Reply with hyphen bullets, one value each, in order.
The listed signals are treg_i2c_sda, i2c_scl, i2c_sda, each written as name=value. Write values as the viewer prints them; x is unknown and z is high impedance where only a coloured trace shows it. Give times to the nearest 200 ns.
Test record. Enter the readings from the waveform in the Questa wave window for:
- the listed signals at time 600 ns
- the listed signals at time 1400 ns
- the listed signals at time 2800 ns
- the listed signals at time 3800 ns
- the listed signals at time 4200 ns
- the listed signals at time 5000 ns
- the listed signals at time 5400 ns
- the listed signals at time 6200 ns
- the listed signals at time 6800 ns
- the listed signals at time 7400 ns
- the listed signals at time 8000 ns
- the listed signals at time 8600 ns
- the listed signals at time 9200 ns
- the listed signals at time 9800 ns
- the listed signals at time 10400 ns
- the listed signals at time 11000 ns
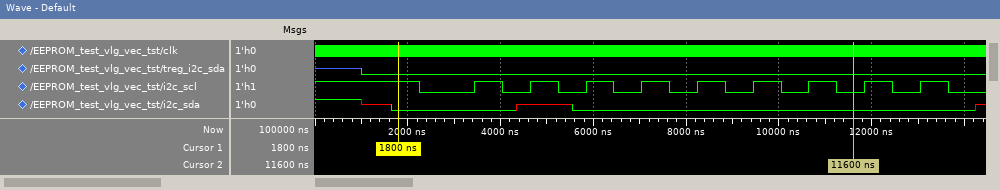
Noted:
- treg_i2c_sda=z, i2c_scl=1, i2c_sda=1
- treg_i2c_sda=0, i2c_scl=1, i2c_sda=x
- treg_i2c_sda=0, i2c_scl=0, i2c_sda=0
- treg_i2c_sda=0, i2c_scl=1, i2c_sda=0
- treg_i2c_sda=0, i2c_scl=0, i2c_sda=0
- treg_i2c_sda=0, i2c_scl=1, i2c_sda=x
- treg_i2c_sda=0, i2c_scl=0, i2c_sda=x
- treg_i2c_sda=0, i2c_scl=1, i2c_sda=0
- treg_i2c_sda=0, i2c_scl=0, i2c_sda=0
- treg_i2c_sda=0, i2c_scl=1, i2c_sda=0
- treg_i2c_sda=0, i2c_scl=0, i2c_sda=0
- treg_i2c_sda=0, i2c_scl=1, i2c_sda=0
- treg_i2c_sda=0, i2c_scl=0, i2c_sda=0
- treg_i2c_sda=0, i2c_scl=1, i2c_sda=0
- treg_i2c_sda=0, i2c_scl=0, i2c_sda=0
- treg_i2c_sda=0, i2c_scl=1, i2c_sda=0
